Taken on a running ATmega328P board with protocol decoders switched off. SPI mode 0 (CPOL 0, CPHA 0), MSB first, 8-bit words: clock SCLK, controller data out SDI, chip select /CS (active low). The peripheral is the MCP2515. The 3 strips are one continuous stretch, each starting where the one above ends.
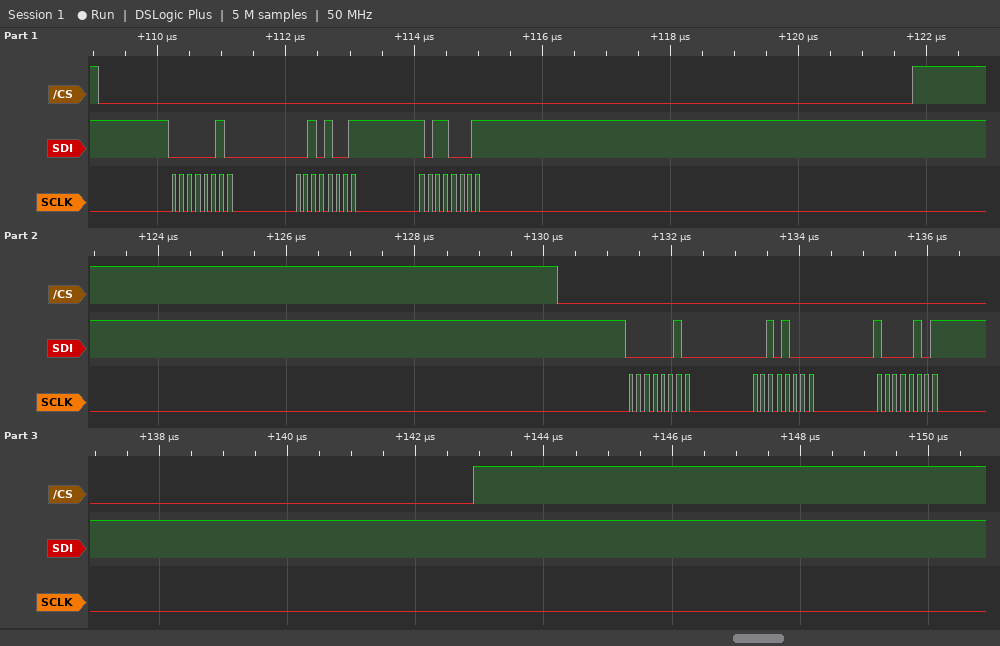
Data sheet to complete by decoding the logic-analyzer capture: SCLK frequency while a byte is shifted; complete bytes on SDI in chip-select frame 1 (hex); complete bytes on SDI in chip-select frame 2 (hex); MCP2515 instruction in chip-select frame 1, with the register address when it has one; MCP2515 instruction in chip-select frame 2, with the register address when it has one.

8 MHz
02 29 B1
02 28 85
WRITE 0x29
WRITE 0x28
